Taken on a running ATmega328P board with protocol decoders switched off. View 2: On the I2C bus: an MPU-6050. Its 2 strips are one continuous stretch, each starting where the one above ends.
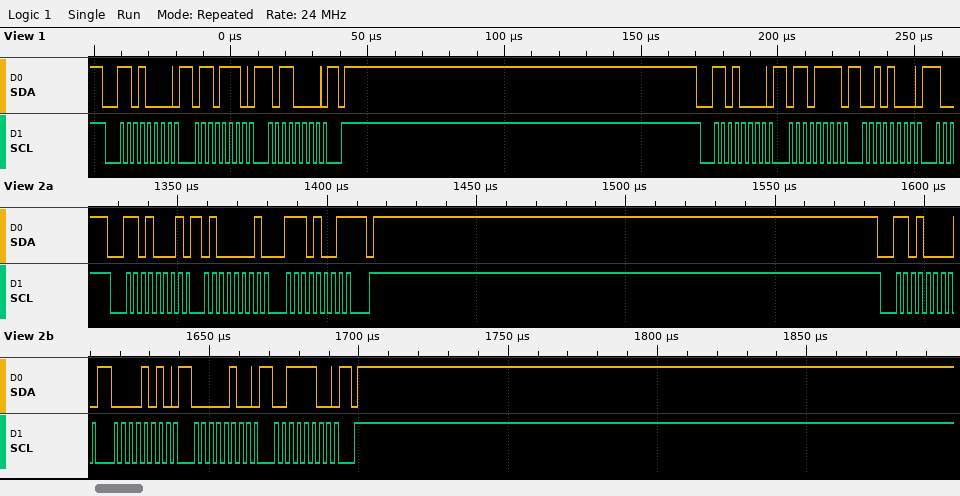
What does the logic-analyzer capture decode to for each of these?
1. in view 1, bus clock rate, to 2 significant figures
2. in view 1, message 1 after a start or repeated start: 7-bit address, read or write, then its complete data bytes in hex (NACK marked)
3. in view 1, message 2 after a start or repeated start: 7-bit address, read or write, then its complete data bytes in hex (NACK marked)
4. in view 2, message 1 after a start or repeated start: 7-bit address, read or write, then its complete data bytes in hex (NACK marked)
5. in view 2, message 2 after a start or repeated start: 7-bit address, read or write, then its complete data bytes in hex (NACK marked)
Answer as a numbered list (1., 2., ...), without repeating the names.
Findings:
1. 400 kHz
2. 0x68 write: 6E B0
3. 0x68 write: 6F 28
4. 0x68 read: 41 E9 NACK
5. 0x68 write: 0A 04 3C
